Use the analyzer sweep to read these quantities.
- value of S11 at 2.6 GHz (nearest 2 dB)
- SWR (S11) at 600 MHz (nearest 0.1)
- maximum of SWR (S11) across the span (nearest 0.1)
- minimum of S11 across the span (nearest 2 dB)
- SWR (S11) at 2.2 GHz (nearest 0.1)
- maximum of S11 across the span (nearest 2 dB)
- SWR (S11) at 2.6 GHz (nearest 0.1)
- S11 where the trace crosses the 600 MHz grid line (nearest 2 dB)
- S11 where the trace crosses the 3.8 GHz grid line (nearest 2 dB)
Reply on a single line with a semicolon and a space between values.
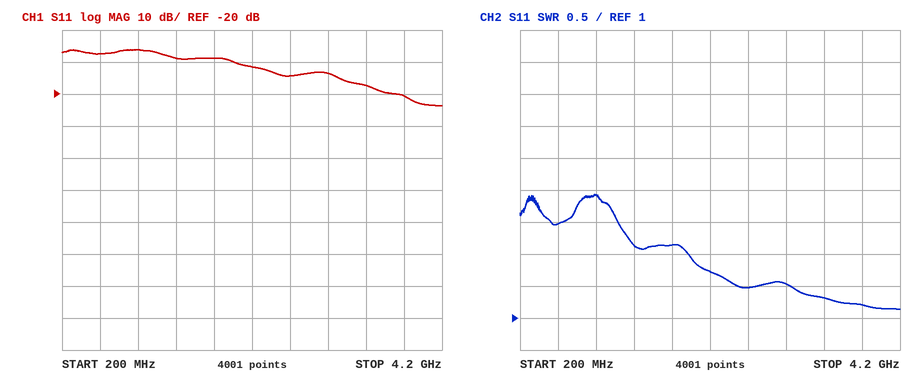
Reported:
-14 dB; 2.5; 2.9; -24 dB; 1.7; -6 dB; 1.5; -8 dB; -20 dB
